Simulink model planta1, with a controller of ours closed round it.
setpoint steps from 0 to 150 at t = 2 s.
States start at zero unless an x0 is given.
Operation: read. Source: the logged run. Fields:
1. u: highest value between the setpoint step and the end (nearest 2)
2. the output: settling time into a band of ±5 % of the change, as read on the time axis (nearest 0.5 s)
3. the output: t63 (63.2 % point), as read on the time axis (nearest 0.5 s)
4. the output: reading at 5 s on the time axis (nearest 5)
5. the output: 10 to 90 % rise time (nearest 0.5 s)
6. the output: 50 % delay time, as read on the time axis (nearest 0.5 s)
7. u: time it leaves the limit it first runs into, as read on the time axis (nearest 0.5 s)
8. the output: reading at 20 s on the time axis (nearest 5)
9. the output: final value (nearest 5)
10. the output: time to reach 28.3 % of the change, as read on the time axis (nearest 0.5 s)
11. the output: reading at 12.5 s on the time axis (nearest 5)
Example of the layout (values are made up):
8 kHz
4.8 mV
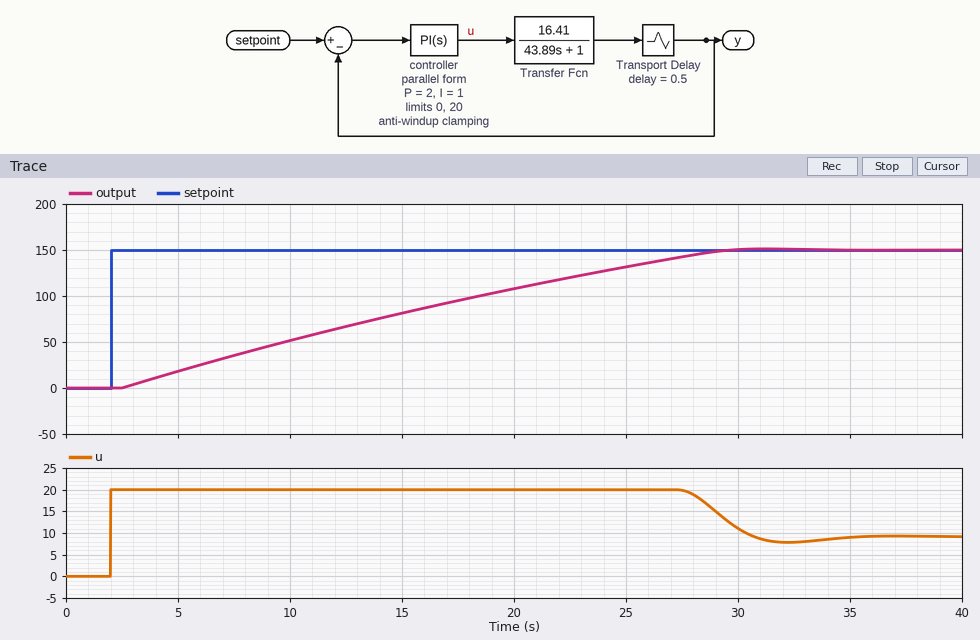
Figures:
20
27.5 s
17.5 s
20
21.0 s
14.0 s
27.5 s
110
150
8.5 s
65
